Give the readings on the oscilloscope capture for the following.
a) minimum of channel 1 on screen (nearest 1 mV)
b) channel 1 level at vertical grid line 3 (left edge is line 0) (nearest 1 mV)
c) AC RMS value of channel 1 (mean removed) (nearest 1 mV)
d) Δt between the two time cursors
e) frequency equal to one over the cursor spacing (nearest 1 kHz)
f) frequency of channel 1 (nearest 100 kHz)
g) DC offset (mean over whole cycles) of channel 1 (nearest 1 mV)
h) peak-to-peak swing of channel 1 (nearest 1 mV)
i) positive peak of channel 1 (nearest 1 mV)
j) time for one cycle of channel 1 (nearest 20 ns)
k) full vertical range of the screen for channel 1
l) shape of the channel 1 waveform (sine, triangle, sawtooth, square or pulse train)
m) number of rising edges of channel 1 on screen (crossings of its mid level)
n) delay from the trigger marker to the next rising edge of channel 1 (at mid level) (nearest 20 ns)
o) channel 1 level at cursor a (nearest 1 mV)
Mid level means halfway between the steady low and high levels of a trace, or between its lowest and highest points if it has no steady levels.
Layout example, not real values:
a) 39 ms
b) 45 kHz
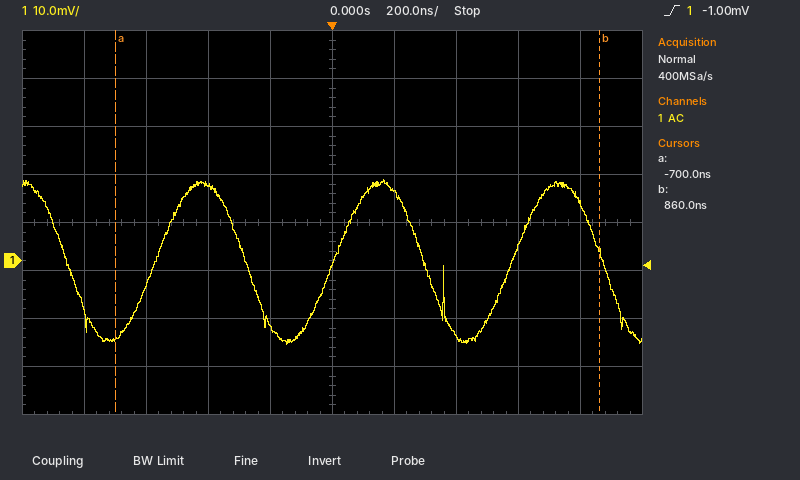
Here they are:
a) -17 mV
b) 16 mV
c) 12 mV
d) 1.56 µs
e) 641 kHz
f) 1.7 MHz
g) 0 mV
h) 34 mV
i) 17 mV
j) 580 ns
k) 80 mV
l) sine
m) 3
n) 580 ns
o) -16 mV
